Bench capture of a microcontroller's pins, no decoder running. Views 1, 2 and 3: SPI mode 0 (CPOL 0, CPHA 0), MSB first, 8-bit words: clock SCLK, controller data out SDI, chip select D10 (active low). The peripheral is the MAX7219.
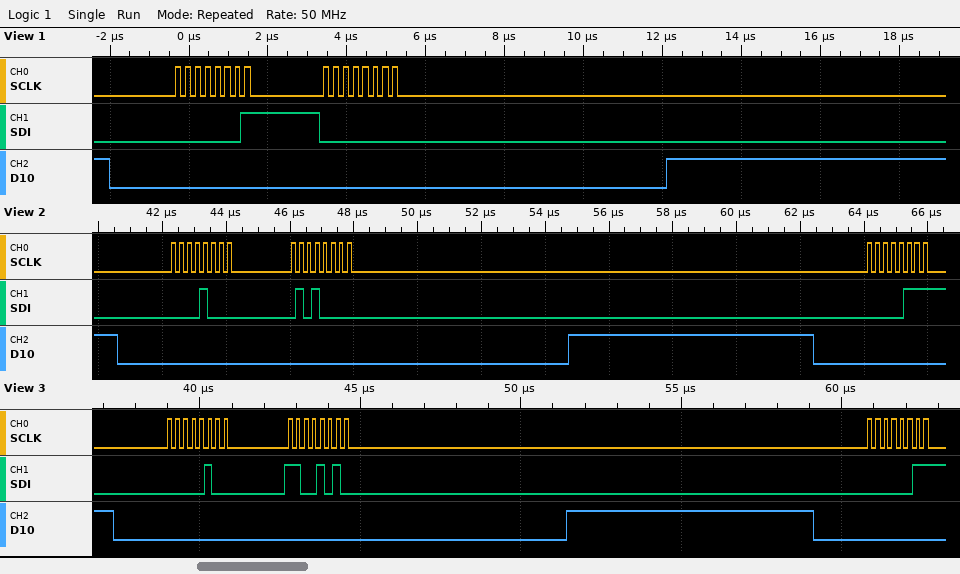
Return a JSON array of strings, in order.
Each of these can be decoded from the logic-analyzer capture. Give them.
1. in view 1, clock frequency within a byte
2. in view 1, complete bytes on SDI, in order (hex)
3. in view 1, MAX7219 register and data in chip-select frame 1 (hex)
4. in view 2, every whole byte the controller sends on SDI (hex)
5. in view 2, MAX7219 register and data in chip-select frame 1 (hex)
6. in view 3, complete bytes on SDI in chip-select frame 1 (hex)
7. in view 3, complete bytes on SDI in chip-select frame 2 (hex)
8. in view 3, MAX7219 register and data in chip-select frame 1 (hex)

["4 MHz", "01 00", "register 0x1, data 0x00", "08 50 07", "register 0x8, data 0x50", "04 CA", "03", "register 0x4, data 0xCA"]
